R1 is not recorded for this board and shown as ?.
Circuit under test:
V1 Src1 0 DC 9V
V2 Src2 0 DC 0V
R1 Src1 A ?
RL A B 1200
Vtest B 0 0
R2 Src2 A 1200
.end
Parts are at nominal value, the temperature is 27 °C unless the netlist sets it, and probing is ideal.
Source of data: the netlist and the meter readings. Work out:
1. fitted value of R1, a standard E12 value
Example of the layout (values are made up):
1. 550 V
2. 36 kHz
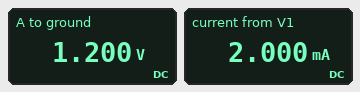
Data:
1. 3.9 kΩ
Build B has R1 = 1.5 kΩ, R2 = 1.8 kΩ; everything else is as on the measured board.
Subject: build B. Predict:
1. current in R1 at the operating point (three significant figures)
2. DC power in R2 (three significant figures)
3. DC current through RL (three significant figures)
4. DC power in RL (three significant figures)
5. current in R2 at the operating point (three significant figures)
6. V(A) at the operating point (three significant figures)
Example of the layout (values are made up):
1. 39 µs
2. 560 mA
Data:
1. 4.05 mA
2. 4.73 mW
3. 2.43 mA
4. 7.10 mW
5. 1.62 mA
6. 2.92 V
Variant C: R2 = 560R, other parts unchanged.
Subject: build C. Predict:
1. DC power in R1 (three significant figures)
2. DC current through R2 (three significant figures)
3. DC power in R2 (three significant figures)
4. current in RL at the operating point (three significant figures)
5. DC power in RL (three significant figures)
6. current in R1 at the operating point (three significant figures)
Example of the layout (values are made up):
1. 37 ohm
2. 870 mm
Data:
1. 17.2 mW
2. 1.43 mA
3. 1.15 mW
4. 669 µA
5. 537 µW
6. 2.10 mA
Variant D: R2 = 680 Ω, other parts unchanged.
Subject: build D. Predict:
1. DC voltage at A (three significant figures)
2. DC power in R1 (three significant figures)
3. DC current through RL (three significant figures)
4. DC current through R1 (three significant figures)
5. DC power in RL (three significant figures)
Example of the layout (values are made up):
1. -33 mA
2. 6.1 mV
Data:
1. 901 mV
2. 16.8 mW
3. 751 µA
4. 2.08 mA
5. 677 µW
